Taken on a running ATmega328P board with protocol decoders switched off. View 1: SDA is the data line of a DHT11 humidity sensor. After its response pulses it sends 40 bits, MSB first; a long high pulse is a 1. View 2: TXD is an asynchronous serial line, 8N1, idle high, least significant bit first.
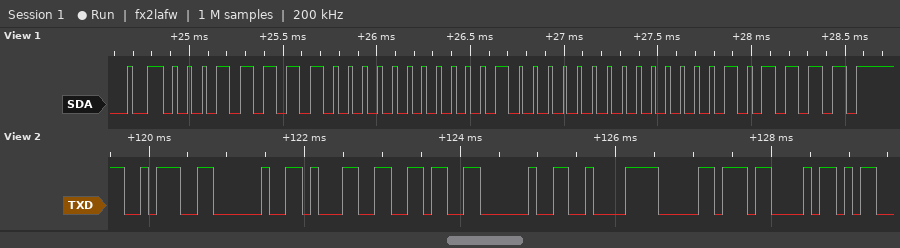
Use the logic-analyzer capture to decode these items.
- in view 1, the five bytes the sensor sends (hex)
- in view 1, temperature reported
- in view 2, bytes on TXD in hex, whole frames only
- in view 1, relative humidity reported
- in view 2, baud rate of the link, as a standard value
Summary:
1F 00 10 00 2F
16.0 °C
3A 20 31 36 20 C2 B0 43
31 %
9600 baud
